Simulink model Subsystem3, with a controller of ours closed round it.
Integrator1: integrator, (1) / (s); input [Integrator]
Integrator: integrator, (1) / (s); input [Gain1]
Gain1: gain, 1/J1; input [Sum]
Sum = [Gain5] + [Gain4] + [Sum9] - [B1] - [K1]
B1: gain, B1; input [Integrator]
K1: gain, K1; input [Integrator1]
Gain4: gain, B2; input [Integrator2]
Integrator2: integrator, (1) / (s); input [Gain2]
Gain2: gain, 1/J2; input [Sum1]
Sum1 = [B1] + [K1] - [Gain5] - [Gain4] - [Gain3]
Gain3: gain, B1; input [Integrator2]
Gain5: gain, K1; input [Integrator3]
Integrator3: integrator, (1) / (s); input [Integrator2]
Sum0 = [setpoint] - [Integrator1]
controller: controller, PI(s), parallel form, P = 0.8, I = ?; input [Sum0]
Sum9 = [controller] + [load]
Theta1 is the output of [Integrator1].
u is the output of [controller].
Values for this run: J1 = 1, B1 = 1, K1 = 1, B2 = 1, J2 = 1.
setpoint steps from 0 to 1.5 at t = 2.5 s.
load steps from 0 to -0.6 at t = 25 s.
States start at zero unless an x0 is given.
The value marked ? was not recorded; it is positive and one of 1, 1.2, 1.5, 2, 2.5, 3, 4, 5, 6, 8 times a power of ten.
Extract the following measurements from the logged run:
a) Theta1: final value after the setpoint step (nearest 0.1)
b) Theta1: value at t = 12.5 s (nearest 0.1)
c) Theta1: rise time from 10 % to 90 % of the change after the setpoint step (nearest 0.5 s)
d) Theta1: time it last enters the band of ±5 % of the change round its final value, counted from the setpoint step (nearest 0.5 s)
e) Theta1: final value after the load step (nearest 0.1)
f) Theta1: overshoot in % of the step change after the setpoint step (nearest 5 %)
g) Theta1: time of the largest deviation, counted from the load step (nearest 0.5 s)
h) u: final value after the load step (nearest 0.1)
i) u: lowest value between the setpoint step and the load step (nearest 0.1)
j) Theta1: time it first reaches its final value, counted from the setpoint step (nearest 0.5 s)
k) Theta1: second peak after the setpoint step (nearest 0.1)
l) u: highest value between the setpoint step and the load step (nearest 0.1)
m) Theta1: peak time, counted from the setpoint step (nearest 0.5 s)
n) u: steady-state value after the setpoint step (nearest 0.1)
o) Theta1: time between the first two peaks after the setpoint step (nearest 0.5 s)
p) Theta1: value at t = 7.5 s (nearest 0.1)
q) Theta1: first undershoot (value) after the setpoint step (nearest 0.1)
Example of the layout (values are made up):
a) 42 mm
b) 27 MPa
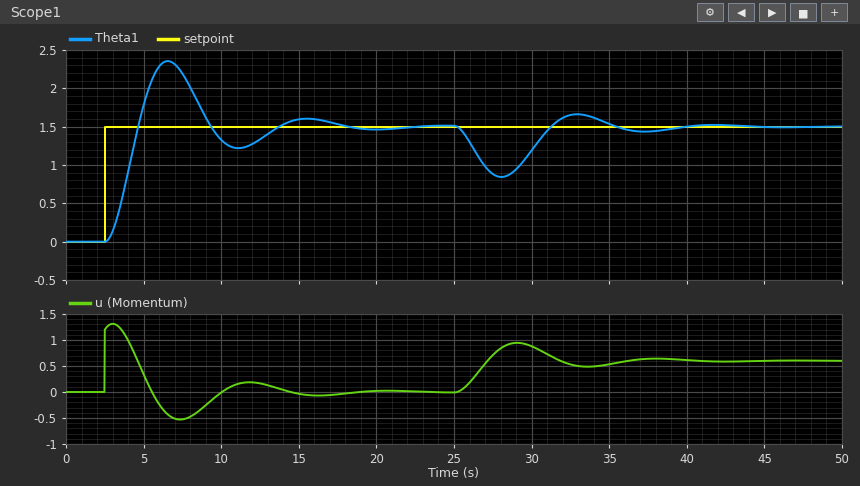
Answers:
a) 1.5
b) 1.3
c) 1.5 s
d) 14.0 s
e) 1.5
f) 55 %
g) 3.0 s
h) 0.6
i) -0.5
j) 2.0 s
k) 1.6
l) 1.3
m) 4.0 s
n) 0.0
o) 9.0 s
p) 2.2
q) 1.2
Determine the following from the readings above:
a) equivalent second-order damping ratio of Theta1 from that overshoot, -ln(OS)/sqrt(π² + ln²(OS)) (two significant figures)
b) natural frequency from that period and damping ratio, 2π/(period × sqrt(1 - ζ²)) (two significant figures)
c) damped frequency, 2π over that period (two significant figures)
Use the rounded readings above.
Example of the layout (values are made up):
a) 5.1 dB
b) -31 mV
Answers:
a) 0.19
b) 0.71 rad/s
c) 0.70 rad/s
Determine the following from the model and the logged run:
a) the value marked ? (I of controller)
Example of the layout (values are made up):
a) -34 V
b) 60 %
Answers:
a) 0.3
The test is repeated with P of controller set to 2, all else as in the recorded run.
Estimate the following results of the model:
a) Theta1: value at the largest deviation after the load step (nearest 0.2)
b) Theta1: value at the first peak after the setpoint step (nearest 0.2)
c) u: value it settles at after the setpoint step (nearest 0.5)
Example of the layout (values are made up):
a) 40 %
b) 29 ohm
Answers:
a) 1.2
b) 2.2
c) 0.0
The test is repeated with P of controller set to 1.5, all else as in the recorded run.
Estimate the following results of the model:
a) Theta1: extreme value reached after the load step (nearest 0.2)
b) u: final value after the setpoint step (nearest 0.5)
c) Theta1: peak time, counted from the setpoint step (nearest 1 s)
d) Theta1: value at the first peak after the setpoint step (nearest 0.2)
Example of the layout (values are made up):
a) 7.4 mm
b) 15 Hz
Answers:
a) 1.0
b) 0.0
c) 3 s
d) 2.2
